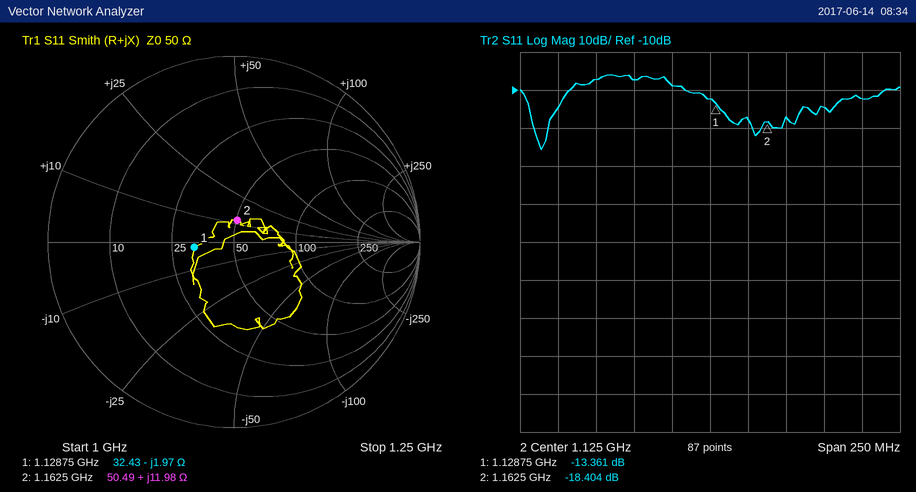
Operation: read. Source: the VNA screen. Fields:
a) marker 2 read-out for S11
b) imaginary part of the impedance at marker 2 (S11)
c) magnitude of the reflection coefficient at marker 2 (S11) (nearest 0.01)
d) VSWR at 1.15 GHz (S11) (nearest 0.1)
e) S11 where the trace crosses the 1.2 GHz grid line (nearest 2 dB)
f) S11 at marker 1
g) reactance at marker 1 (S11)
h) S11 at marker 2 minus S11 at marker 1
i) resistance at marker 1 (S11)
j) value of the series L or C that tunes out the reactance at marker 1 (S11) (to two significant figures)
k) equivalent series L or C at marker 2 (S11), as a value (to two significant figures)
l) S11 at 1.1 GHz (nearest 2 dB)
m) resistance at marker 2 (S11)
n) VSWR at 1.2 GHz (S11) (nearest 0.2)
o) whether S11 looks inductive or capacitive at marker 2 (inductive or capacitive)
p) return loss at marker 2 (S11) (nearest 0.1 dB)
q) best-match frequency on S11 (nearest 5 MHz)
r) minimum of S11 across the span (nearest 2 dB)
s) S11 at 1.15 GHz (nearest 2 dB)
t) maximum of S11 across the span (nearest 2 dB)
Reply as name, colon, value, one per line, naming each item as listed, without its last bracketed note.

marker 2 read-out for S11: -18.404 dB
imaginary part of the impedance at marker 2: +11.98 Ω
magnitude of the reflection coefficient at marker 2 (S11): 0.12
VSWR at 1.15 GHz (S11): 1.3
S11 where the trace crosses the 1.2 GHz grid line: -14 dB
S11 at marker 1: -13.361 dB
reactance at marker 1: -1.97 Ω
S11 at marker 2 minus S11 at marker 1: -5.043 dB
resistance at marker 1: 32.43 Ω
value of the series L or C that tunes out the reactance at marker 1 (S11): 280 pH
equivalent series L or C at marker 2 (S11), as a value: 1.6 nH
S11 at 1.1 GHz: -8 dB
resistance at marker 2: 50.49 Ω
VSWR at 1.2 GHz (S11): 1.4
whether S11 looks inductive or capacitive at marker 2: inductive
return loss at marker 2 (S11): 18.5 dB
best-match frequency on S11: 1.015 GHz
minimum of S11 across the span: -26 dB
S11 at 1.15 GHz: -18 dB
maximum of S11 across the span: -6 dB
